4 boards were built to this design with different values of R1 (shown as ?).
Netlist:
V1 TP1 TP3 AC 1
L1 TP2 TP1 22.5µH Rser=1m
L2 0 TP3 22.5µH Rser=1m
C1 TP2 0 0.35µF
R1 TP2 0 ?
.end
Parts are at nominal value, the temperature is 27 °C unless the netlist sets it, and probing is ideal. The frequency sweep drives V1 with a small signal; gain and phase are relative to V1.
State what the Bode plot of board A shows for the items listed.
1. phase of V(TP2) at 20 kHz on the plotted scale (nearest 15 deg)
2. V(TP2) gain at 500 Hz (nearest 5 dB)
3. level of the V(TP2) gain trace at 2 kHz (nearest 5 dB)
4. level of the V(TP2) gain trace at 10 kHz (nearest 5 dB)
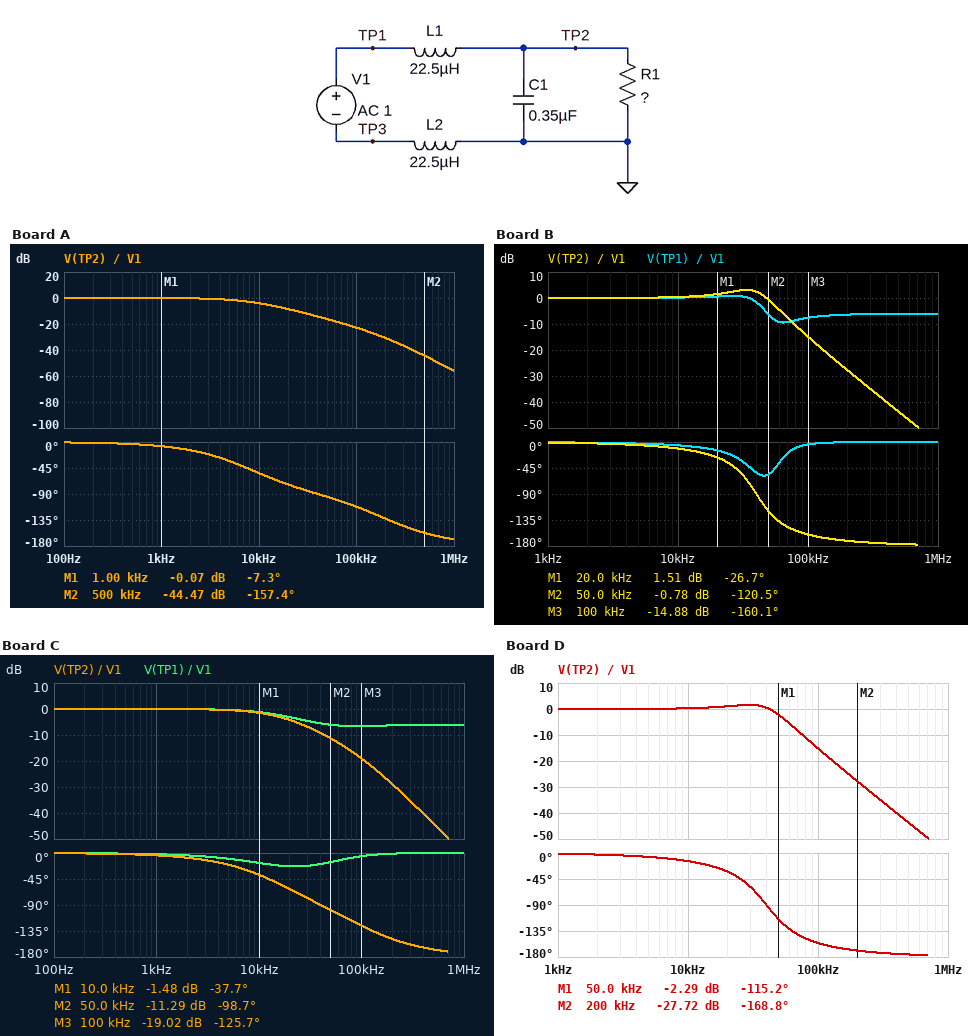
-75 deg
0 dB
0 dB
-5 dB
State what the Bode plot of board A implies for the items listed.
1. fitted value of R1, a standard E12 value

2.2 Ω
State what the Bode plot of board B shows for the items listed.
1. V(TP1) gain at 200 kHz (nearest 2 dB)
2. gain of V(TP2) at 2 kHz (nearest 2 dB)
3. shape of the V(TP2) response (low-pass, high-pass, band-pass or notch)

-6 dB
0 dB
low-pass
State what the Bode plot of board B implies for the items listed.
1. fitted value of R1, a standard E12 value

15 Ω
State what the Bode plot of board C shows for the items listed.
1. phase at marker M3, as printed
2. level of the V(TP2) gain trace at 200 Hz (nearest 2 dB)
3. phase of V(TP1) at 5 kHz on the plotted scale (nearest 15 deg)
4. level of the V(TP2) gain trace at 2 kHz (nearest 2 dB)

-125.7 deg
0 dB
-15 deg
0 dB
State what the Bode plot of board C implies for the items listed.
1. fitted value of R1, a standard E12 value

3.9 Ω
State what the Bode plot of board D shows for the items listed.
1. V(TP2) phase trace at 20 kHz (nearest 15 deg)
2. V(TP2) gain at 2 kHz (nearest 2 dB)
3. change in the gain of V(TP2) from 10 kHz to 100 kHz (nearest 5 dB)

-30 deg
0 dB
-15 dB
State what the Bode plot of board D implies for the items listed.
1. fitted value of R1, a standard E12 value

12 Ω
